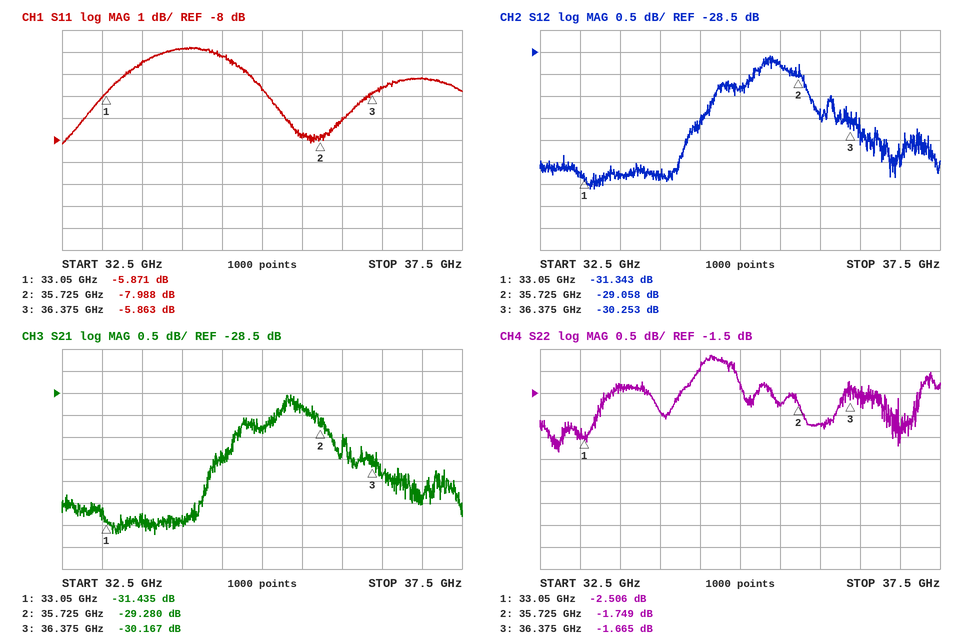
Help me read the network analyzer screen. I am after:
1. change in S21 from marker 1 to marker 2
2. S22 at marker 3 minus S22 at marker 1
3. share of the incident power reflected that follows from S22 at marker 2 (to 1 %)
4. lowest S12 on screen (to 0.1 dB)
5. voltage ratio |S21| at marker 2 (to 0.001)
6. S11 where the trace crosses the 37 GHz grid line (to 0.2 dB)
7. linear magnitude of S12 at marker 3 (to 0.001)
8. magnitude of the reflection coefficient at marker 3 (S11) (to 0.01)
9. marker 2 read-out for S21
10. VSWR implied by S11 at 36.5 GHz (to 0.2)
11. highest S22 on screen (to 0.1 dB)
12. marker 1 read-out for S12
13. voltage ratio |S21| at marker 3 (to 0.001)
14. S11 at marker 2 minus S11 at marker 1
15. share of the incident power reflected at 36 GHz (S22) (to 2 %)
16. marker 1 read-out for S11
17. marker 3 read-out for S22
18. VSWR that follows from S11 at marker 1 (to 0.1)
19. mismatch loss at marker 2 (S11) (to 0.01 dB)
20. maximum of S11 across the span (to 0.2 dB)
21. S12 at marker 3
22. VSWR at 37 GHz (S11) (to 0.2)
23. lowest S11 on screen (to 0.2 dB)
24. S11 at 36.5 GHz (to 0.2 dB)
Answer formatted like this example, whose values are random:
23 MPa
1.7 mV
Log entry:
2.155 dB
0.841 dB
67 %
-31.6 dB
0.034
-5.2 dB
0.031
0.51
-29.280 dB
3.2
-0.6 dB
-31.343 dB
0.031
-2.117 dB
60 %
-5.871 dB
-1.665 dB
3.1
0.75 dB
-3.8 dB
-30.253 dB
3.4
-8.2 dB
-5.6 dB
